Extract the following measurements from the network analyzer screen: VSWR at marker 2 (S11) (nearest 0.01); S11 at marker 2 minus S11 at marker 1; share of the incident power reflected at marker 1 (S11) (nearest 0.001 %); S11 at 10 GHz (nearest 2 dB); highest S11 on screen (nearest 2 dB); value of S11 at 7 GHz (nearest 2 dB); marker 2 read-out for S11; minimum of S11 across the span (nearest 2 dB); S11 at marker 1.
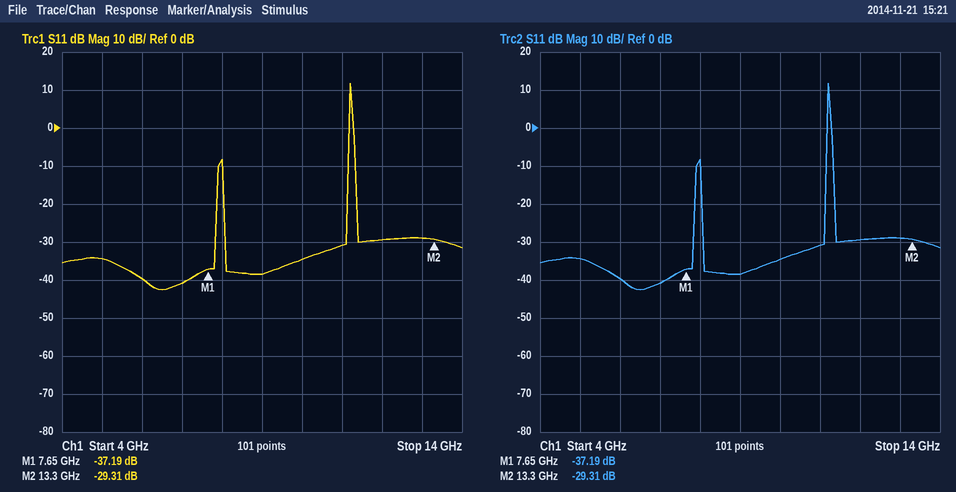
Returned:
1.07
7.88 dB
0.019 %
-34 dB
12 dB
-40 dB
-29.31 dB
-42 dB
-37.19 dB
